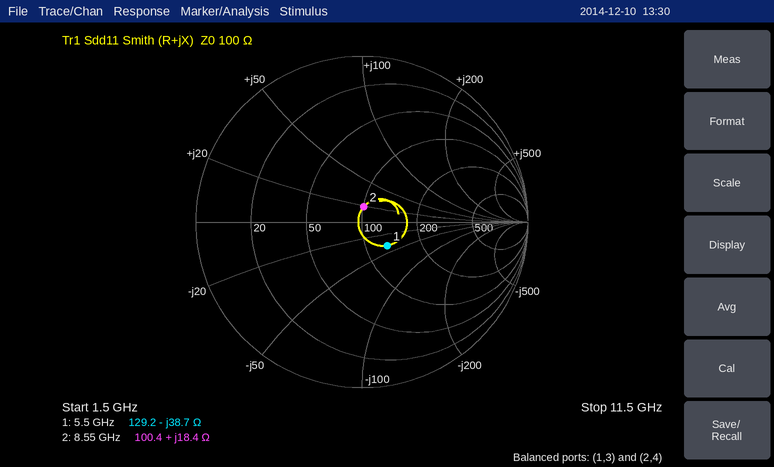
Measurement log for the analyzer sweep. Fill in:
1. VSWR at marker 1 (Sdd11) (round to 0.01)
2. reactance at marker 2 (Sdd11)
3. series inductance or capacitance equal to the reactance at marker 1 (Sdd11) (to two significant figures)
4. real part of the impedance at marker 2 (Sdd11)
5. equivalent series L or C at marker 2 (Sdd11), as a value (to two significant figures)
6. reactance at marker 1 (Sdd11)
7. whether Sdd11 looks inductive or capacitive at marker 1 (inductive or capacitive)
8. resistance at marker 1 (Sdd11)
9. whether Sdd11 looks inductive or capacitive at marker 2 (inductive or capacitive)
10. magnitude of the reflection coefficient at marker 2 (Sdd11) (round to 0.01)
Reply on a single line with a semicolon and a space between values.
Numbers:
1.53; +18.4 Ω; 750 fF; 100.4 Ω; 340 pH; -38.7 Ω; capacitive; 129.2 Ω; inductive; 0.09
